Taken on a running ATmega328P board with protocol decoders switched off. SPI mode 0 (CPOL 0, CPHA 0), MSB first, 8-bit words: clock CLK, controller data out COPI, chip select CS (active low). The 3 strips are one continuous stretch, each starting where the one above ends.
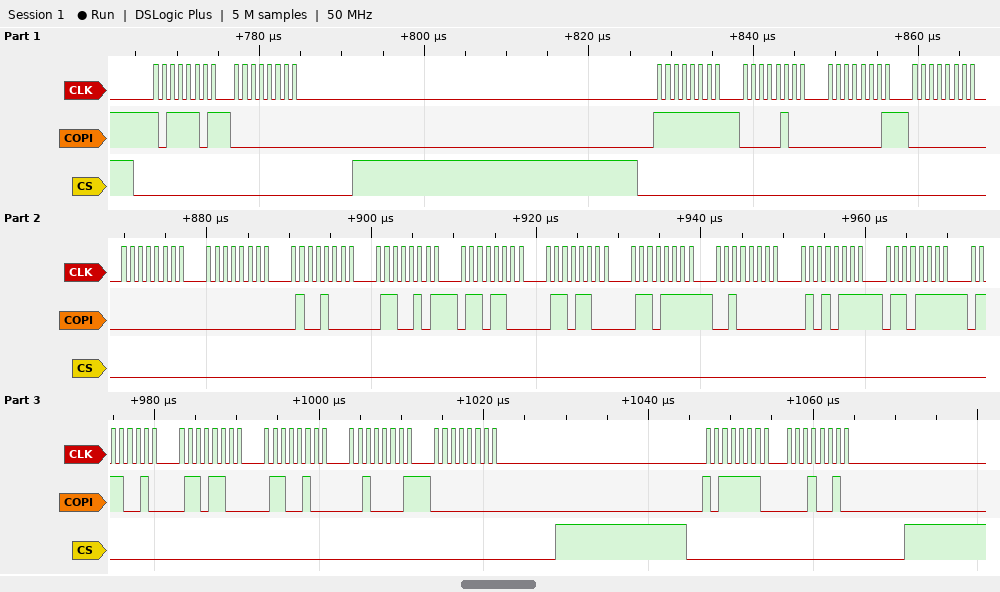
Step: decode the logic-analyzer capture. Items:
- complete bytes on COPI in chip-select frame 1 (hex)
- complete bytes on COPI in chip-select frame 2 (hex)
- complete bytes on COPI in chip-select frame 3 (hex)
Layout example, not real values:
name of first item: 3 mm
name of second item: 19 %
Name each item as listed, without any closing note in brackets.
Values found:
complete bytes on COPI in chip-select frame 1: BD 00
complete bytes on COPI in chip-select frame 2: FF 04 01 00 00 00 48 65 6C 6C 6F 20 57 6F 72 6C 64 21 00
complete bytes on COPI in chip-select frame 3: BE 12
